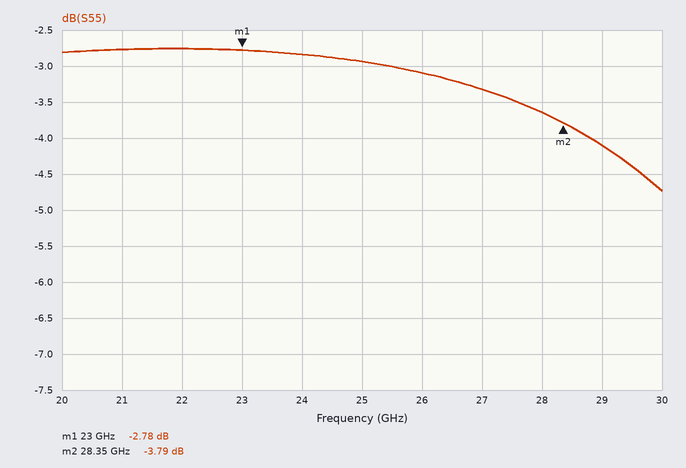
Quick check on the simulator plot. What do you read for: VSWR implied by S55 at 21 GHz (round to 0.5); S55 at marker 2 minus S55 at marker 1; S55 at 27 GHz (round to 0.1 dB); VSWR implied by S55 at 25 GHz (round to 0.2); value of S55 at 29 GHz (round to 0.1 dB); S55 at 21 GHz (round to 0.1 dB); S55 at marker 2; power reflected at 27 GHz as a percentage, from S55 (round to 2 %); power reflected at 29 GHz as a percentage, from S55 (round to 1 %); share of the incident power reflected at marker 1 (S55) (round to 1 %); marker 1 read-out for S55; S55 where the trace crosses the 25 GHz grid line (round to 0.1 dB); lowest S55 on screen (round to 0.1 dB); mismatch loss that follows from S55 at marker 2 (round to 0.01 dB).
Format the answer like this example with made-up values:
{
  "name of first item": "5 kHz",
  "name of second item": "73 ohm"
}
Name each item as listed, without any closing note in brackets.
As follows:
{
  "VSWR implied by S55 at 21 GHz": "6.5",
  "S55 at marker 2 minus S55 at marker 1": "-1.01 dB",
  "S55 at 27 GHz": "-3.3 dB",
  "VSWR implied by S55 at 25 GHz": "6.0",
  "value of S55 at 29 GHz": "-4.1 dB",
  "S55 at 21 GHz": "-2.8 dB",
  "S55 at marker 2": "-3.79 dB",
  "power reflected at 27 GHz as a percentage, from S55": "46 %",
  "power reflected at 29 GHz as a percentage, from S55": "39 %",
  "share of the incident power reflected at marker 1 (S55)": "53 %",
  "marker 1 read-out for S55": "-2.78 dB",
  "S55 where the trace crosses the 25 GHz grid line": "-2.9 dB",
  "lowest S55 on screen": "-4.7 dB",
  "mismatch loss that follows from S55 at marker 2": "2.35 dB"
}
